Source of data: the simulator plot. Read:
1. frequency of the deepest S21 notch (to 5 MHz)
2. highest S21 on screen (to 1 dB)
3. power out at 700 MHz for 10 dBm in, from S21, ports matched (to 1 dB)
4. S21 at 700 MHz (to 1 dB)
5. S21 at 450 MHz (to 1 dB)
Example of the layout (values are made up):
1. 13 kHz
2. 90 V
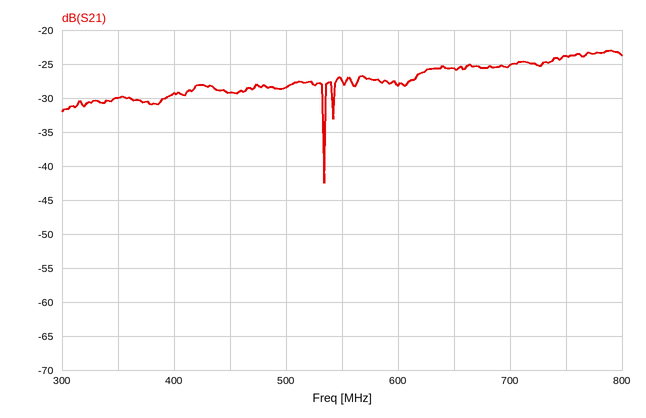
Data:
1. 535 MHz
2. -23 dB
3. -15 dBm
4. -25 dB
5. -29 dB
